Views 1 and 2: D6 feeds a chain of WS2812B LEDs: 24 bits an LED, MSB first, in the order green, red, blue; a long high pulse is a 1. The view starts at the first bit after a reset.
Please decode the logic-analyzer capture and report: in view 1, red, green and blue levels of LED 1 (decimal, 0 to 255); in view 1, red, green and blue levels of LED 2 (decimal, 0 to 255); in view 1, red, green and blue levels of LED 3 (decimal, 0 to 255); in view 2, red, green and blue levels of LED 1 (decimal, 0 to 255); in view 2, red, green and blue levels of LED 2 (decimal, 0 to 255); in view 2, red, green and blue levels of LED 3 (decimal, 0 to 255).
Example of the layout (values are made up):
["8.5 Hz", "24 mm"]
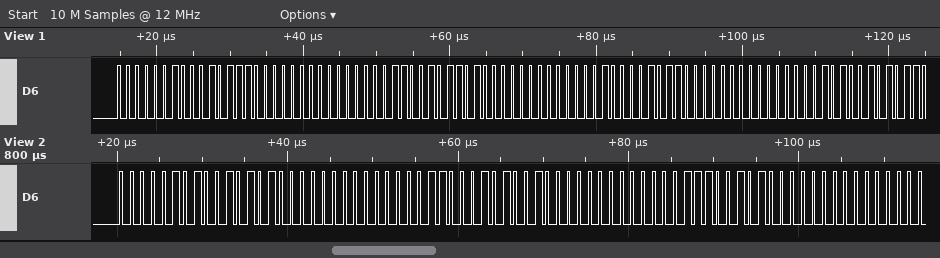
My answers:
["46, 2, 0", "45, 3, 0", "44, 4, 0", "42, 5, 0", "41, 6, 0", "40, 7, 0"]
